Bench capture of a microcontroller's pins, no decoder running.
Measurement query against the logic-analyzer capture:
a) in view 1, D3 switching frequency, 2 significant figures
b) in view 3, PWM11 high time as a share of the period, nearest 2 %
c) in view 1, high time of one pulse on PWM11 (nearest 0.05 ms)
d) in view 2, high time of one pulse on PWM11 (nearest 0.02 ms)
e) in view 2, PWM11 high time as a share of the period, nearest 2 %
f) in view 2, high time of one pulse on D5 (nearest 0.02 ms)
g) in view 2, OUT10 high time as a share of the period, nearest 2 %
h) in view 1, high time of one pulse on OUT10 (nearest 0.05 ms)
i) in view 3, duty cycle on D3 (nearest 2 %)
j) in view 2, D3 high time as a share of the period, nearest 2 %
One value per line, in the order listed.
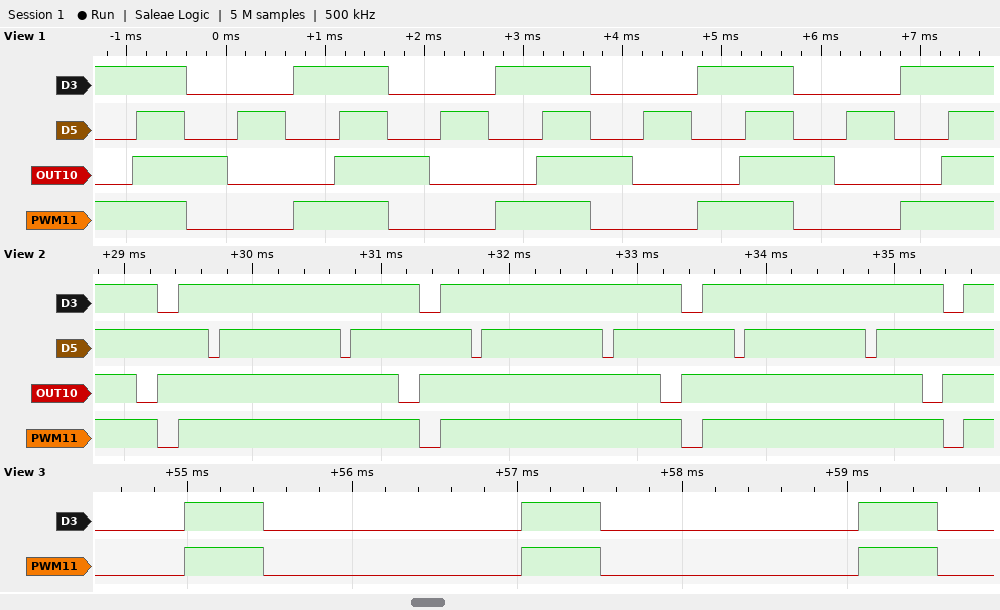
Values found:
490 Hz
24 %
0.95 ms
1.88 ms
92 %
0.94 ms
92 %
0.95 ms
24 %
92 %
